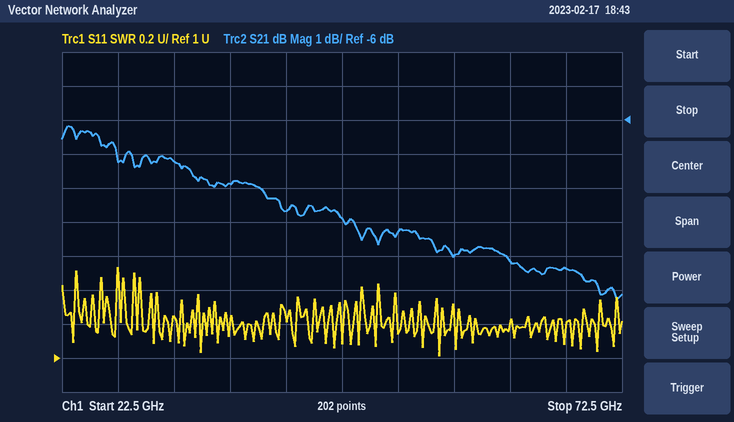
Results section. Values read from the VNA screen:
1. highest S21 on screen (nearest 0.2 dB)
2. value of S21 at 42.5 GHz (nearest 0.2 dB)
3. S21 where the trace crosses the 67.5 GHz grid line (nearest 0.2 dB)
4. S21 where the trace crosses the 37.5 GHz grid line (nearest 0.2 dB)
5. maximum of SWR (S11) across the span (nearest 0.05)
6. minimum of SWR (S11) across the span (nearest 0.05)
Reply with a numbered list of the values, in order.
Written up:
1. -6.2 dB
2. -8.6 dB
3. -10.4 dB
4. -7.8 dB
5. 1.55
6. 1.00
